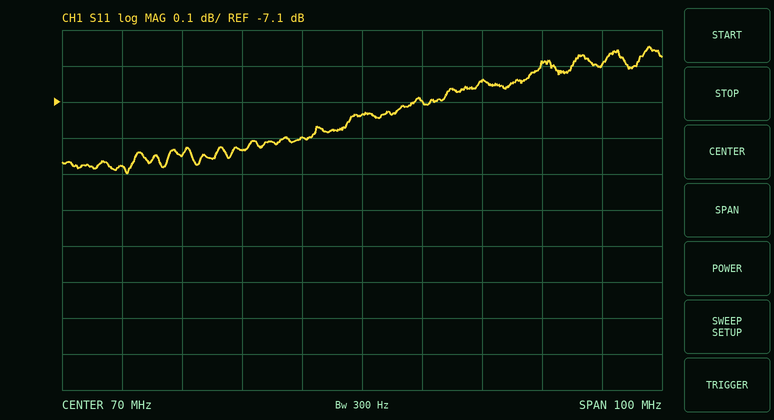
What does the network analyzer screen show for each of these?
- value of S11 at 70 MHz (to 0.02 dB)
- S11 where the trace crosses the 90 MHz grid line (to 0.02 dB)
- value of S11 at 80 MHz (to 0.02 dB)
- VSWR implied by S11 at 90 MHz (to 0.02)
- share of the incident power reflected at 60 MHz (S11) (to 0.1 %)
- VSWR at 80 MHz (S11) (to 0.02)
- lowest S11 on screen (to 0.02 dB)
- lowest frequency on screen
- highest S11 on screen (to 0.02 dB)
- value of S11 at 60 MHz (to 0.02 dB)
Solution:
-7.14 dB
-7.04 dB
-7.10 dB
2.60
19.1 %
2.58
-7.30 dB
20 MHz
-6.94 dB
-7.20 dB
